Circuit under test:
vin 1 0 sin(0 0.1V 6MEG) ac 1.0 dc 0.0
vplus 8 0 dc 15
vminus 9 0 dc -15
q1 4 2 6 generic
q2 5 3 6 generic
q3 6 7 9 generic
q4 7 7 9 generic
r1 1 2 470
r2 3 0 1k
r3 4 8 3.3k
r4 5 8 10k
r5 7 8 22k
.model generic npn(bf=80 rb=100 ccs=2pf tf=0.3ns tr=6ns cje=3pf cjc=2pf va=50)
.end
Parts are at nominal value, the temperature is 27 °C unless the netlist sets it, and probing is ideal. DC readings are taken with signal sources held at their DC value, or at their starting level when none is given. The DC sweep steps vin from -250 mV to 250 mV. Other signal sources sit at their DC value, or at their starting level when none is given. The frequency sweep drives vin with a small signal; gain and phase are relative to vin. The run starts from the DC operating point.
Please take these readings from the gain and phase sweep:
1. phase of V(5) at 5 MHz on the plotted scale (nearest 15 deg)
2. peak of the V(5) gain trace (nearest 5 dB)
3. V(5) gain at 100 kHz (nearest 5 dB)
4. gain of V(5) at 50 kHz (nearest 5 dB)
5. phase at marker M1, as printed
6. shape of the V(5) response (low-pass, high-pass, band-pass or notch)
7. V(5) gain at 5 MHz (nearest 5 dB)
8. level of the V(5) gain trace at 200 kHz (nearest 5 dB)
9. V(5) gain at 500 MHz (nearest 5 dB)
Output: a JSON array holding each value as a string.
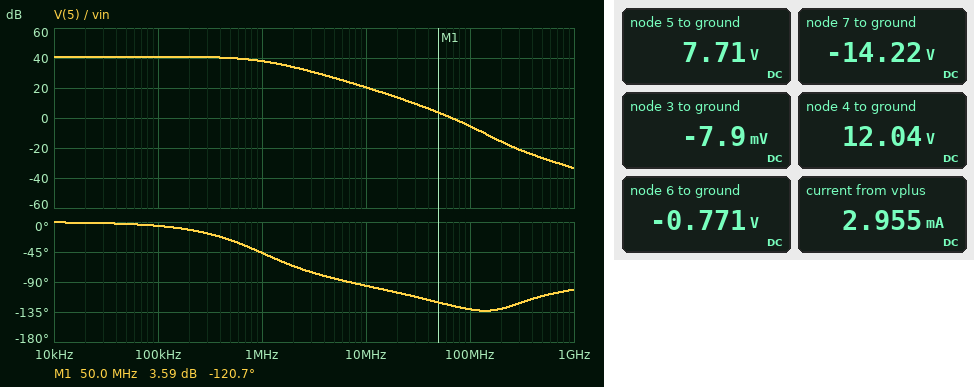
["-90 deg", "40 dB", "40 dB", "40 dB", "-120.7 deg", "low-pass", "25 dB", "40 dB", "-25 dB"]
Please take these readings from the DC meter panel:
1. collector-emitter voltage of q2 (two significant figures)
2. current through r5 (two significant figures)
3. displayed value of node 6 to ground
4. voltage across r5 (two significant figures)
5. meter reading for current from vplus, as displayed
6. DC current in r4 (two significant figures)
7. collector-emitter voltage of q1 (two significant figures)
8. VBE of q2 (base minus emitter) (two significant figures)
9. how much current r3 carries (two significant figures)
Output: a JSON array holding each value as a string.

["8.5 V", "1.3 mA", "-0.771 V", "29 V", "2.955 mA", "730 µA", "13 V", "760 mV", "900 µA"]
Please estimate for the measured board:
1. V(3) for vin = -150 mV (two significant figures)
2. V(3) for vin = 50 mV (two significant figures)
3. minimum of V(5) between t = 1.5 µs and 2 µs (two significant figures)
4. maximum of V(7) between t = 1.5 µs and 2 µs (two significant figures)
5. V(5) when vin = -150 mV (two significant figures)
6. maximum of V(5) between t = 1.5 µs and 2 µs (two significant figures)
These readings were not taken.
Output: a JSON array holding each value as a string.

["-38 mV", "-2.5 mV", "5.9 V", "-14 V", "-710 mV", "9.5 V"]
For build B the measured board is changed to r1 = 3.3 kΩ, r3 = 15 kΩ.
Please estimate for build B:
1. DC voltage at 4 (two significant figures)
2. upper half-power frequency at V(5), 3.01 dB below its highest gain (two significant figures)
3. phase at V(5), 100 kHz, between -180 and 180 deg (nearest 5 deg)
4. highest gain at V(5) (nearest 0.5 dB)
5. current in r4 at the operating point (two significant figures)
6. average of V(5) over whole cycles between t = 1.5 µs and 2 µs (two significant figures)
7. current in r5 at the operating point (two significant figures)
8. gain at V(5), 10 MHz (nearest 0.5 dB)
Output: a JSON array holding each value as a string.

["5.5 V", "320 kHz", "-15 deg", "37.0 dB", "990 µA", "5.1 V", "1.3 mA", "9.5 dB"]
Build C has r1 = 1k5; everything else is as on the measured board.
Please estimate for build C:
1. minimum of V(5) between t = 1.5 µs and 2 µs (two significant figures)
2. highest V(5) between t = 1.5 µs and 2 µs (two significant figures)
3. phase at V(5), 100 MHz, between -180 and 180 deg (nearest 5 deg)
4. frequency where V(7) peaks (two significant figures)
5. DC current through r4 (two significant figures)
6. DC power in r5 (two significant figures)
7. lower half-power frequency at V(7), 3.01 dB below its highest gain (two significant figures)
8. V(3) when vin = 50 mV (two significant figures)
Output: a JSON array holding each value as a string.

["5.4 V", "8.2 V", "-145 deg", "120 MHz", "820 µA", "39 mW", "38 MHz", "-3.6 mV"]
